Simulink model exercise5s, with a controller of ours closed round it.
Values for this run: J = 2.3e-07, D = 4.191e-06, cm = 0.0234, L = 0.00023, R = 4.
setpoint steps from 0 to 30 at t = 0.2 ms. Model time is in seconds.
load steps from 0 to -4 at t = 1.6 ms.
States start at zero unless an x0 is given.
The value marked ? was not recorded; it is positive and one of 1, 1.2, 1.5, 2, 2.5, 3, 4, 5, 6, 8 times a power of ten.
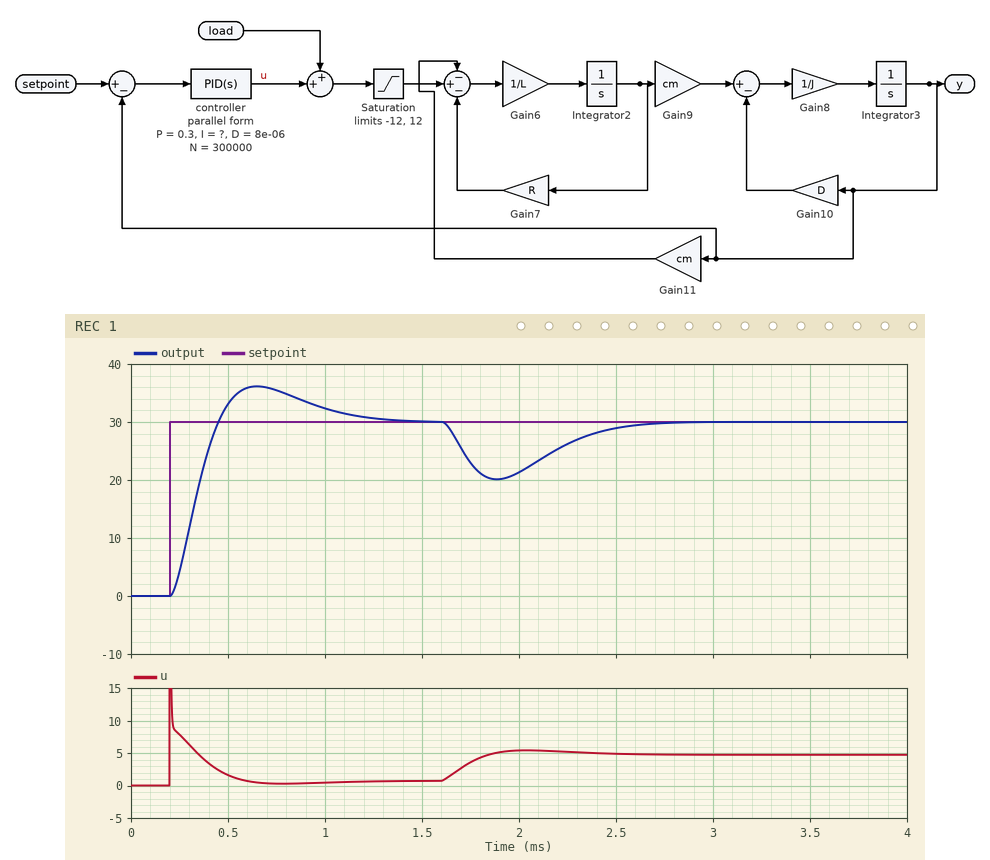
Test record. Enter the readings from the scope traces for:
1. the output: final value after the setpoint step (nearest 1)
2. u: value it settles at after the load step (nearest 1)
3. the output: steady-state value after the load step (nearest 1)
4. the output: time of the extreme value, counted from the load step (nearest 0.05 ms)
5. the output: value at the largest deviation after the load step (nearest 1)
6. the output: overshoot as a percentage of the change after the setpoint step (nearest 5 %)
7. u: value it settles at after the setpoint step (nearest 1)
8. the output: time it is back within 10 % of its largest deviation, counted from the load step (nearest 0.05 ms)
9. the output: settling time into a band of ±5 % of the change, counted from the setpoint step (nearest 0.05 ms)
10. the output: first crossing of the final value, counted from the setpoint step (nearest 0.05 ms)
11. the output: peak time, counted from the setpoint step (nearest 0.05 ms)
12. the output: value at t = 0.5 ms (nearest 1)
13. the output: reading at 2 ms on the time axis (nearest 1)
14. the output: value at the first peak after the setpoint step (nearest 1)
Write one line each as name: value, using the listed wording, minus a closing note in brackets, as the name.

the output: final value after the setpoint step: 30
u: value it settles at after the load step: 5
the output: steady-state value after the load step: 30
the output: time of the extreme value, counted from the load step: 0.30 ms
the output: value at the largest deviation after the load step: 20
the output: overshoot as a percentage of the change after the setpoint step: 20 %
u: value it settles at after the setpoint step: 1
the output: time it is back within 10 % of its largest deviation, counted from the load step: 0.90 ms
the output: settling time into a band of ±5 % of the change, counted from the setpoint step: 0.90 ms
the output: first crossing of the final value, counted from the setpoint step: 0.25 ms
the output: peak time, counted from the setpoint step: 0.45 ms
the output: value at t = 0.5 ms: 33
the output: reading at 2 ms on the time axis: 21
the output: value at the first peak after the setpoint step: 36
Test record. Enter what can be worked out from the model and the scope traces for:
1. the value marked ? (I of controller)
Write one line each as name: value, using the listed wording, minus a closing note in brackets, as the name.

the value marked ?: 800
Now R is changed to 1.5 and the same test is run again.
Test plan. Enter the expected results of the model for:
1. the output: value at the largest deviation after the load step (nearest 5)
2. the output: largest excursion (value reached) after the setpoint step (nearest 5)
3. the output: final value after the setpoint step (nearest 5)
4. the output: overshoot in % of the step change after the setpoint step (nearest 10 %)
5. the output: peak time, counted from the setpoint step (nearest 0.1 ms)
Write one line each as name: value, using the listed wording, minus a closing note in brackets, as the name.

the output: value at the largest deviation after the load step: 15
the output: largest excursion (value reached) after the setpoint step: 40
the output: final value after the setpoint step: 30
the output: overshoot in % of the step change after the setpoint step: 40 %
the output: peak time, counted from the setpoint step: 0.3 ms
